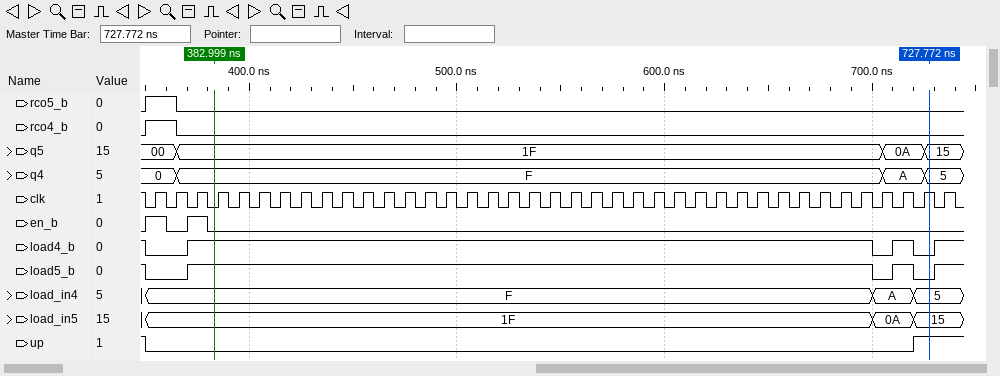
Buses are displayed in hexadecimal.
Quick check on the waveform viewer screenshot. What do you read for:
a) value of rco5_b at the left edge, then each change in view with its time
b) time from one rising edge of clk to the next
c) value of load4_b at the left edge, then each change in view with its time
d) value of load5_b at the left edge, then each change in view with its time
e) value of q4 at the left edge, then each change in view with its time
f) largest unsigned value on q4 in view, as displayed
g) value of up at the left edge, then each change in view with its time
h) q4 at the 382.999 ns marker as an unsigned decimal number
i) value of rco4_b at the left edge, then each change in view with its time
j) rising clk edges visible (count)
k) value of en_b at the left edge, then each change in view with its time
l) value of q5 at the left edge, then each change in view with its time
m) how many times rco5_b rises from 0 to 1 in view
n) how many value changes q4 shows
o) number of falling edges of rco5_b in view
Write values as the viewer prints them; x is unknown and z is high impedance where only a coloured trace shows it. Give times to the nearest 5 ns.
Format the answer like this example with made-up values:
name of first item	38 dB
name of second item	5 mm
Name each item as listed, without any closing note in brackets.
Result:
value of rco5_b at the left edge, then each change in view with its time	0, 1 at 350 ns, 0 at 365 ns
time from one rising edge of clk to the next	10 ns
value of load4_b at the left edge, then each change in view with its time	1, 0 at 350 ns, 1 at 370 ns, 0 at 700 ns, 1 at 710 ns, 0 at 720 ns, 1 at 730 ns
value of load5_b at the left edge, then each change in view with its time	1, 0 at 350 ns, 1 at 370 ns, 0 at 700 ns, 1 at 710 ns, 0 at 720 ns, 1 at 730 ns
value of q4 at the left edge, then each change in view with its time	0, F at 365 ns, A at 705 ns, 5 at 725 ns
largest unsigned value on q4 in view, as displayed	F
value of up at the left edge, then each change in view with its time	1, 0 at 350 ns, 1 at 720 ns
q4 at the 382.999 ns marker as an unsigned decimal number	15
value of rco4_b at the left edge, then each change in view with its time	0, 1 at 350 ns, 0 at 365 ns
rising clk edges visible	39
value of en_b at the left edge, then each change in view with its time	0, 1 at 350 ns, 0 at 360 ns, 1 at 370 ns, 0 at 380 ns
value of q5 at the left edge, then each change in view with its time	00, 1F at 365 ns, 0A at 705 ns, 15 at 725 ns
how many times rco5_b rises from 0 to 1 in view	1
how many value changes q4 shows	3
number of falling edges of rco5_b in view	1
